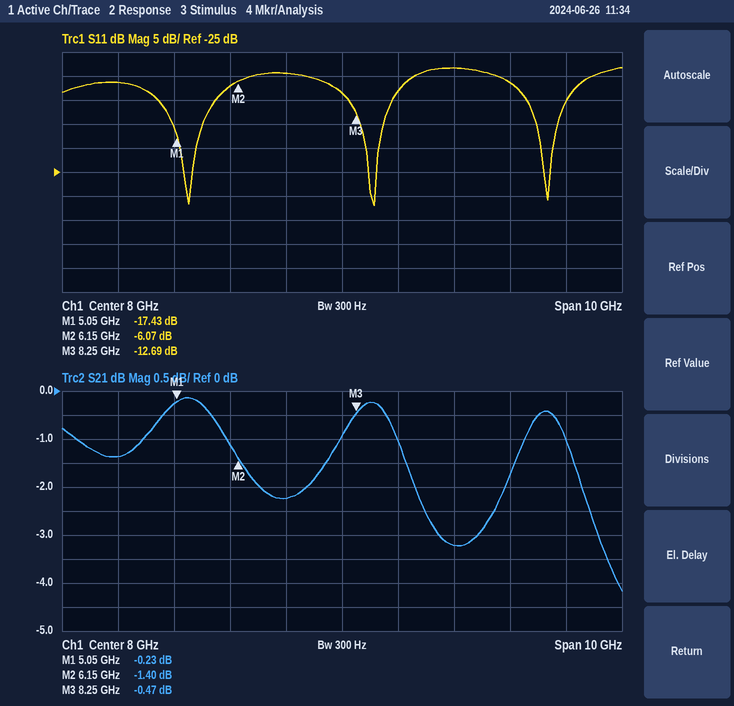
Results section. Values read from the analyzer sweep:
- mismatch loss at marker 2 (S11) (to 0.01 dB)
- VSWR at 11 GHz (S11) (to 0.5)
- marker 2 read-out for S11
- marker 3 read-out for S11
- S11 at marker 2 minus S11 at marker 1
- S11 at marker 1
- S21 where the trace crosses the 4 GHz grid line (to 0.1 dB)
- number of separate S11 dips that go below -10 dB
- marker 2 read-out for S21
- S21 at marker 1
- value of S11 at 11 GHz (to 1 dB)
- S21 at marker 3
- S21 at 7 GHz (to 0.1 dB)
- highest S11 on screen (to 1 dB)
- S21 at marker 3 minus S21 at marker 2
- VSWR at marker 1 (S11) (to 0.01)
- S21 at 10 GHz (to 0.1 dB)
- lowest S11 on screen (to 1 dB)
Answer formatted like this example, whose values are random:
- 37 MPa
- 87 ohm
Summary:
- 1.23 dB
- 3.0
- -6.07 dB
- -12.69 dB
- 11.36 dB
- -17.43 dB
- -1.4 dB
- 3
- -1.40 dB
- -0.23 dB
- -6 dB
- -0.47 dB
- -2.2 dB
- -3 dB
- 0.93 dB
- 1.31
- -3.2 dB
- -32 dB
